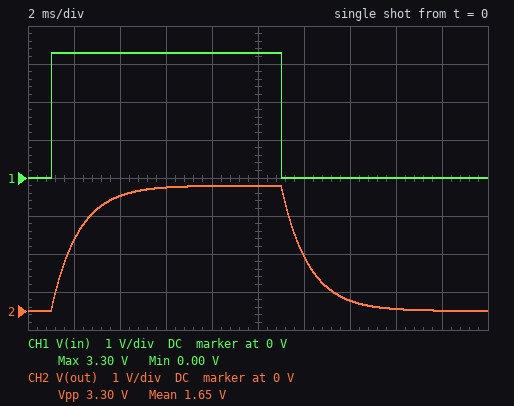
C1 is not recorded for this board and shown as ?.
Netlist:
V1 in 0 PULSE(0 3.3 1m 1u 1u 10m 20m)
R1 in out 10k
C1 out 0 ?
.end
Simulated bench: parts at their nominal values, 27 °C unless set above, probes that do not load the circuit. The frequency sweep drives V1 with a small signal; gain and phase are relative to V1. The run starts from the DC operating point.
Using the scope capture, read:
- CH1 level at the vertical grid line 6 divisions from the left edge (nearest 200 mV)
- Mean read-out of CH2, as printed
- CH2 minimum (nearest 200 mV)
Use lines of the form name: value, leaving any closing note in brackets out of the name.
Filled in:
CH1 level at the vertical grid line 6 divisions from the left edge: 0 V
Mean read-out of CH2, as printed: 1.65 V
CH2 minimum: 0 V
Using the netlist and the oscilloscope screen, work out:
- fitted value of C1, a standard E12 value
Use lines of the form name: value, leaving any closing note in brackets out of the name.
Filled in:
fitted value of C1, a standard E12 value: 120 nF
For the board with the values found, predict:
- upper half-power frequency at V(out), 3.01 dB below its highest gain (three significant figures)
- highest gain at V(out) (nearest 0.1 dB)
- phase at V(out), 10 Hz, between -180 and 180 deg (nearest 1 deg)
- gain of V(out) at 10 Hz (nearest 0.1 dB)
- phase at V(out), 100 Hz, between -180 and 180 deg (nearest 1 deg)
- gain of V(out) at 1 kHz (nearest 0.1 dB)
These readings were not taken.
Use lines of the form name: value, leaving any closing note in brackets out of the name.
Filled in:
upper half-power frequency at V(out), 3.01 dB below its highest gain: 133 Hz
highest gain at V(out): 0 dB
phase at V(out), 10 Hz, between -180 and 180 deg: -4 deg
gain of V(out) at 10 Hz: 0 dB
phase at V(out), 100 Hz, between -180 and 180 deg: -37 deg
gain of V(out) at 1 kHz: -17.6 dB
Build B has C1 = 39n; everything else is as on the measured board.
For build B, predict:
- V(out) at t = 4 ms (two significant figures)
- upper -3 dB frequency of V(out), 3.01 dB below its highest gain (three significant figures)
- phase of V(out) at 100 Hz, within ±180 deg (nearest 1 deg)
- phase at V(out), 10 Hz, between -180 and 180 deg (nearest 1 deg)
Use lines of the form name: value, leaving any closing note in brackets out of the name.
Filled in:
V(out) at t = 4 ms: 3.3 V
upper -3 dB frequency of V(out), 3.01 dB below its highest gain: 408 Hz
phase of V(out) at 100 Hz, within ±180 deg: -14 deg
phase at V(out), 10 Hz, between -180 and 180 deg: -1 deg
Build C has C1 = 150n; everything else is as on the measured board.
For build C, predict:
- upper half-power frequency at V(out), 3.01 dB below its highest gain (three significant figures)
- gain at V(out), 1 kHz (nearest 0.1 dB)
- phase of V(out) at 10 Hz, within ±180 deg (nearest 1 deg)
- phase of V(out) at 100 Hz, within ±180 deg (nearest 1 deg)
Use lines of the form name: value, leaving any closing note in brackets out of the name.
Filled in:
upper half-power frequency at V(out), 3.01 dB below its highest gain: 106 Hz
gain at V(out), 1 kHz: -19.5 dB
phase of V(out) at 10 Hz, within ±180 deg: -5 deg
phase of V(out) at 100 Hz, within ±180 deg: -43 deg
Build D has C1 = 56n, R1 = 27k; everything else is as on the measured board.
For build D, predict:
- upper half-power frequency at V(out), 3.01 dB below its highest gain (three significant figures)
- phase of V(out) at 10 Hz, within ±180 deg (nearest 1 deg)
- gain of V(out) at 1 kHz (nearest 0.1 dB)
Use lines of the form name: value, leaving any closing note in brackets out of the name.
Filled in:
upper half-power frequency at V(out), 3.01 dB below its highest gain: 105 Hz
phase of V(out) at 10 Hz, within ±180 deg: -5 deg
gain of V(out) at 1 kHz: -19.6 dB
